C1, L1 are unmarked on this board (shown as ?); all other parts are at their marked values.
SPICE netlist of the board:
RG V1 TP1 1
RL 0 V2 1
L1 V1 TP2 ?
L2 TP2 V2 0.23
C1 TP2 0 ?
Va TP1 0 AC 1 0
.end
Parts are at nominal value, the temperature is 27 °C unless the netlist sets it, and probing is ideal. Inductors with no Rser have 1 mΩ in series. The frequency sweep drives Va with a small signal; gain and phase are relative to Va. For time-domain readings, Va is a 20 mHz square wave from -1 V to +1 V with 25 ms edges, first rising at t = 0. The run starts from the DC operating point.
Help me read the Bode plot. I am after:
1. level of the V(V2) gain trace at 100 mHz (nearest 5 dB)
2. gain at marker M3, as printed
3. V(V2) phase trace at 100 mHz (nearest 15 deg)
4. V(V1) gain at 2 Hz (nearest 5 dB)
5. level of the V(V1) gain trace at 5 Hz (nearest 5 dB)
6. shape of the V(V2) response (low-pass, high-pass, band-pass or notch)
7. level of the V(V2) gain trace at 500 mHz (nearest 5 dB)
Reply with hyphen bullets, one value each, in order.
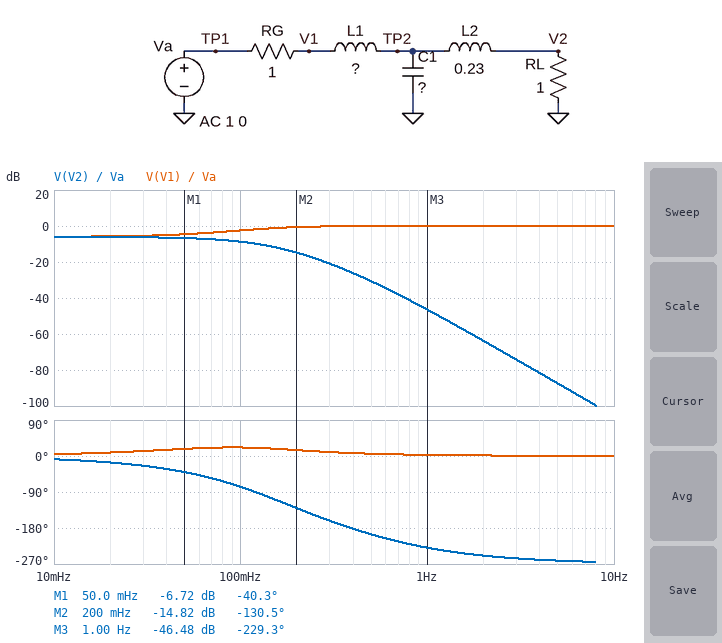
- -10 dB
- -46.48 dB
- -75 deg
- 0 dB
- 0 dB
- low-pass
- -30 dB
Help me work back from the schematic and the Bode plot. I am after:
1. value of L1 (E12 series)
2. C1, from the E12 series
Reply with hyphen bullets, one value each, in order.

- 3.3 H
- 1 F
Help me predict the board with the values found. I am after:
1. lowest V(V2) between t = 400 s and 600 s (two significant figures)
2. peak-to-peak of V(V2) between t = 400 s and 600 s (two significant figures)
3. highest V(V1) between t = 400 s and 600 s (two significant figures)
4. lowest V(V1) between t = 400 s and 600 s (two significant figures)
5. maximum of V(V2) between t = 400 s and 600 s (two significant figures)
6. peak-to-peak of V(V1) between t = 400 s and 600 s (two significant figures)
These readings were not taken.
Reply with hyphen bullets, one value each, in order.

- -500 mV
- 1.0 V
- 1.5 V
- -1.5 V
- 500 mV
- 3.0 V
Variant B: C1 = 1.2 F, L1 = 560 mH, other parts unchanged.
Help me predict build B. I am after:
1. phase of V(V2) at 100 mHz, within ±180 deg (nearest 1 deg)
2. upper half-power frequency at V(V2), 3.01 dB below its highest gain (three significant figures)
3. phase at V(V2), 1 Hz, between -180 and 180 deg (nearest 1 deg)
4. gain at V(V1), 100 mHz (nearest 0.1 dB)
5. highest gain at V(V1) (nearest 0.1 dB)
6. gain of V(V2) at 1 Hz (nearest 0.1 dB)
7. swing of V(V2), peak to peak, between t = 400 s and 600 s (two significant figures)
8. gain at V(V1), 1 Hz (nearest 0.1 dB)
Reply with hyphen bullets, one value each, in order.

- -37 deg
- 281 mHz
- 144 deg
- -7.4 dB
- 0 dB
- -32.8 dB
- 1.1 V
- -0.4 dB
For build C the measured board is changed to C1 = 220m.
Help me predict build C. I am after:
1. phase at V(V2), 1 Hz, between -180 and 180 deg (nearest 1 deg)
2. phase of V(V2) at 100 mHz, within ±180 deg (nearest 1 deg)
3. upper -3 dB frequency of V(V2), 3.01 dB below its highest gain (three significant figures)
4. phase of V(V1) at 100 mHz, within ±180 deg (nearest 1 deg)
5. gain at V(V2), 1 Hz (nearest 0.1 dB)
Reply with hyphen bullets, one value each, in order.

- 148 deg
- -54 deg
- 97.3 mHz
- 18 deg
- -30.6 dB
